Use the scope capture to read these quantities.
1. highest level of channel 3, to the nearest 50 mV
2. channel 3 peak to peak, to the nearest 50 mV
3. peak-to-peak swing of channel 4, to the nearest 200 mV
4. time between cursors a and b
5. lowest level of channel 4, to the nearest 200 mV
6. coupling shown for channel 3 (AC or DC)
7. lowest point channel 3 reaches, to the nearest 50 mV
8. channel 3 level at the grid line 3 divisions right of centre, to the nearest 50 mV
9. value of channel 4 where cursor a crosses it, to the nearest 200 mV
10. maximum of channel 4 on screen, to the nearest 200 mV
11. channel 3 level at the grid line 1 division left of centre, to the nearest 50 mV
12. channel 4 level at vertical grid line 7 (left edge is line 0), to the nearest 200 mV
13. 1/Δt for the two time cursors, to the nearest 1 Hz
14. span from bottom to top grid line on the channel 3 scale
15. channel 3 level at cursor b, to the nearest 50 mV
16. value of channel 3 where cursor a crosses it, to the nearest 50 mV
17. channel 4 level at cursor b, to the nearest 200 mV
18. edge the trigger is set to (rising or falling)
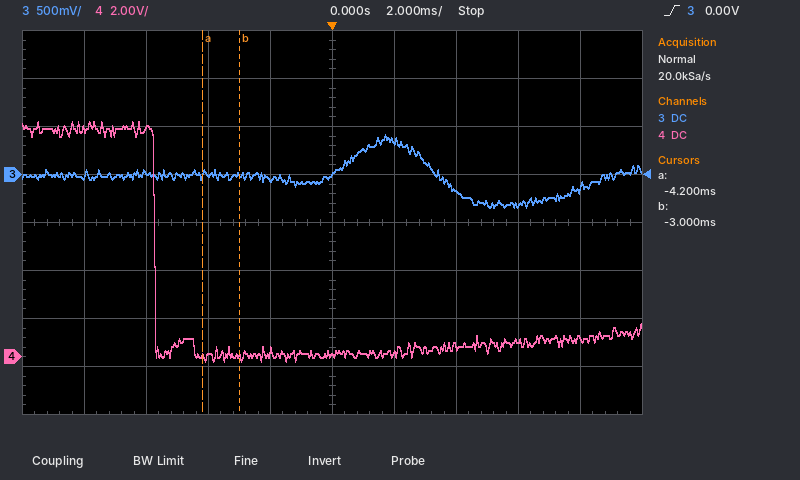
400 mV
750 mV
10.0 V
1.2 ms
-200 mV
DC
-350 mV
-300 mV
0.0 V
9.8 V
-50 mV
400 mV
833 Hz
4 V
0 mV
0 mV
0.0 V
rising
